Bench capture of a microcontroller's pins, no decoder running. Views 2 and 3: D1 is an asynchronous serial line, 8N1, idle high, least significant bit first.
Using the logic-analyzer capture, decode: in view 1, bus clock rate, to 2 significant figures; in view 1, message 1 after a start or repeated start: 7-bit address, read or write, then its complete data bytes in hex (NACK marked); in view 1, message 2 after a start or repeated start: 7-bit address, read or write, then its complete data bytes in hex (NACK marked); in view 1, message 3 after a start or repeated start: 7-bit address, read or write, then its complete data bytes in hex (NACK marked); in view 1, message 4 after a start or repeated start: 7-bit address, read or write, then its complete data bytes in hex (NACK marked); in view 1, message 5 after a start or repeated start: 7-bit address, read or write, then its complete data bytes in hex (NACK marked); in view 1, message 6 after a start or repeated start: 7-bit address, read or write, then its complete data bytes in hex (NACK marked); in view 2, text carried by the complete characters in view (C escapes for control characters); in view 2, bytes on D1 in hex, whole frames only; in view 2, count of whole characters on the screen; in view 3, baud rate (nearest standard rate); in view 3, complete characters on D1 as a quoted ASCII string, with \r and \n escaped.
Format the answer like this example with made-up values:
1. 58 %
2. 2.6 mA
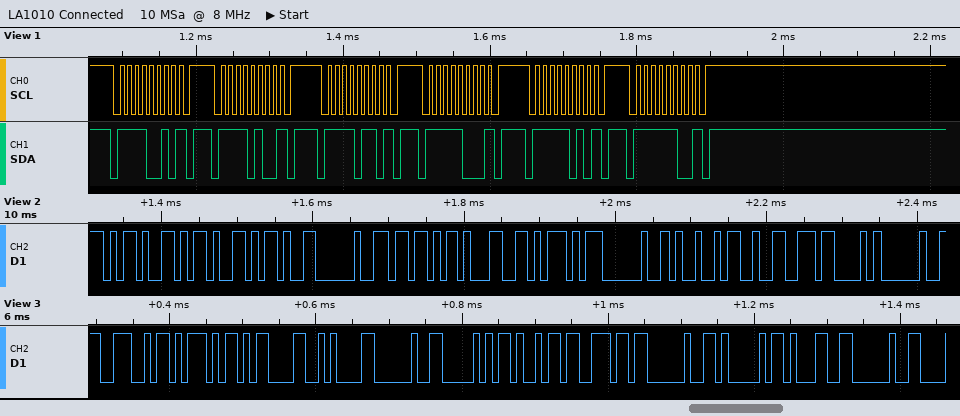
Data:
1. 100 kHz
2. 0x79 write NACK
3. 0x7A write NACK
4. 0x7B write NACK
5. 0x7C write NACK
6. 0x7D write NACK
7. 0x7E write NACK
8. "--- [1] I2C "
9. 0x2D 0x2D 0x2D 0x20 0x5B 0x31 0x5D 0x20 0x49 0x32 0x43 0x20
10. 12
11. 115200 baud
12. "N]\r\n Pin A1 "
